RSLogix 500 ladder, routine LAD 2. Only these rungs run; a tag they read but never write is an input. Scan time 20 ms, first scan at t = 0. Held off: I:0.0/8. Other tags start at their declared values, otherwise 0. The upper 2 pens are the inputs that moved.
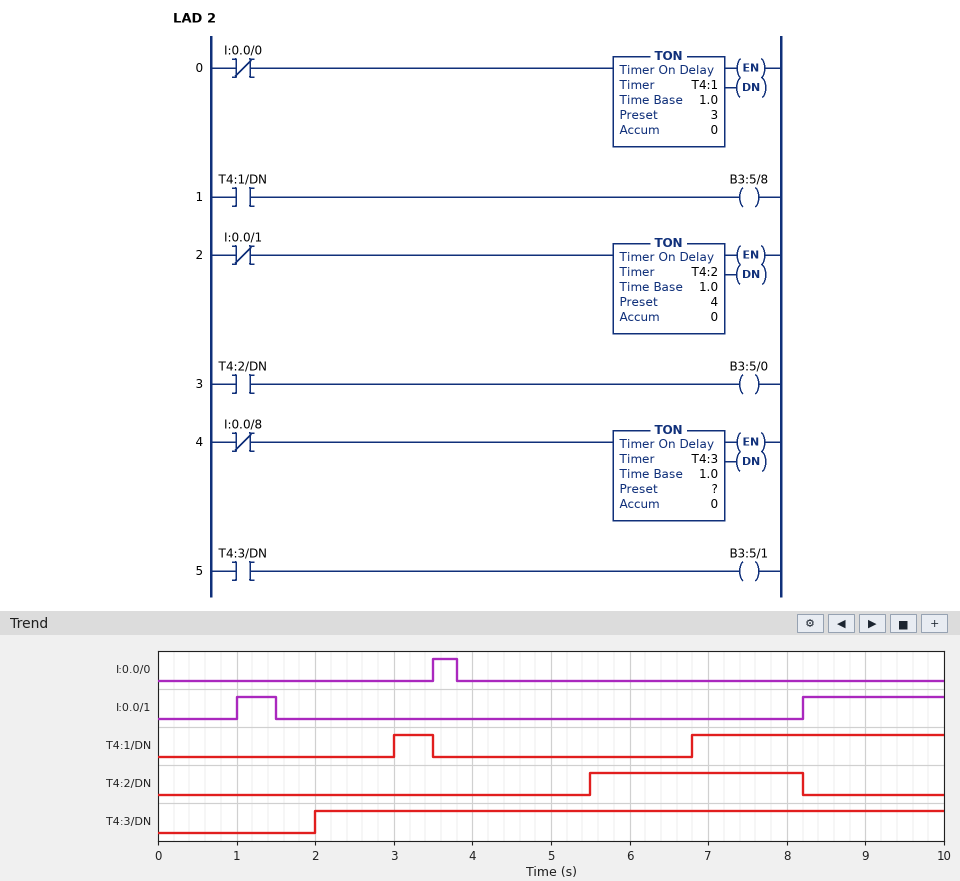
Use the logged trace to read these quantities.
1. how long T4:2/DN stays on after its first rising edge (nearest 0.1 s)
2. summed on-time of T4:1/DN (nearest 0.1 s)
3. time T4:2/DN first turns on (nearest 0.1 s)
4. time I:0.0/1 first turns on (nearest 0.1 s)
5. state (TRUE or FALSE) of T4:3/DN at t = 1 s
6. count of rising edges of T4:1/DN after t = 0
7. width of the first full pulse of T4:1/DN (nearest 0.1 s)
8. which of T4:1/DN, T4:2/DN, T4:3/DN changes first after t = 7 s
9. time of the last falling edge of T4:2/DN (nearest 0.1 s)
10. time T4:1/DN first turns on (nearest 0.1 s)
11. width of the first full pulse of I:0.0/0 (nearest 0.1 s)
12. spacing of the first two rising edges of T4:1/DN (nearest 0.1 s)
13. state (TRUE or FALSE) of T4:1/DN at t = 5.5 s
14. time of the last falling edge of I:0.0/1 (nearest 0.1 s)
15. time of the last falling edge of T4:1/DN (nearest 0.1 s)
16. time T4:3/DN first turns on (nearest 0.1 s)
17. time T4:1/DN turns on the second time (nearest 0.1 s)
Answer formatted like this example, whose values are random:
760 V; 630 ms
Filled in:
2.7 s; 3.7 s; 5.5 s; 1.0 s; FALSE; 2; 0.5 s; T4:2/DN; 8.2 s; 3.0 s; 0.3 s; 3.8 s; FALSE; 1.5 s; 3.5 s; 2.0 s; 6.8 s
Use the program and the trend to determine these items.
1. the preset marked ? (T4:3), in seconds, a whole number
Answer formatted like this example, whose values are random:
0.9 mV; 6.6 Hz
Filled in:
2 s
